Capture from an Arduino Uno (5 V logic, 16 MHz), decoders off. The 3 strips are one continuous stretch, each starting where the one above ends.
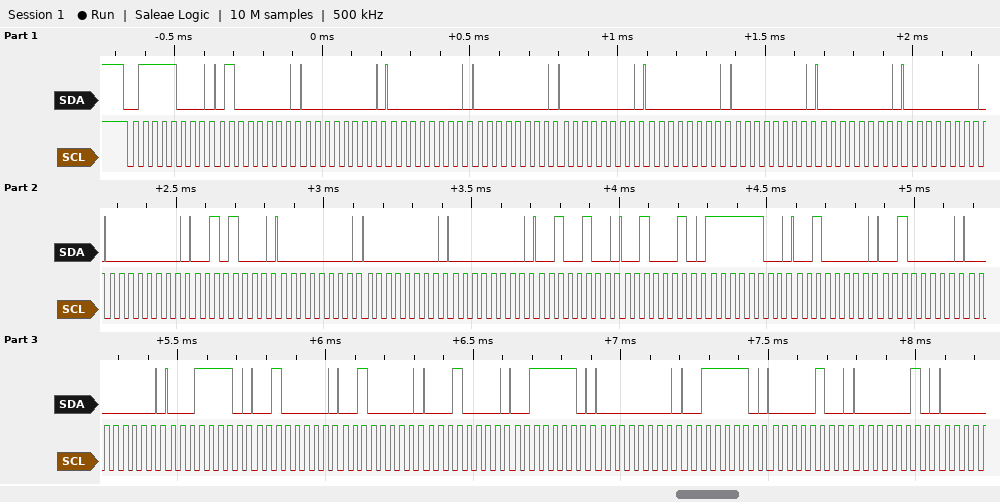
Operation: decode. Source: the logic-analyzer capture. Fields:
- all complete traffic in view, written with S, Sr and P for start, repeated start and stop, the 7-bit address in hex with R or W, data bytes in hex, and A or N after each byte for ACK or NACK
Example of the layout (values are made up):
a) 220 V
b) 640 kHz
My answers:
a) S 3CW A 40 A 00 A 00 A 00 A 00 A 00 A 00 A 00 A 00 A 00 A 28 A 00 A 00 A 00 A 24 A 22 A FC A 20 A 20 A 00 A 1E A 20 A 20 A 10 A 3E A 00 A 3E A 04 A 02 A
